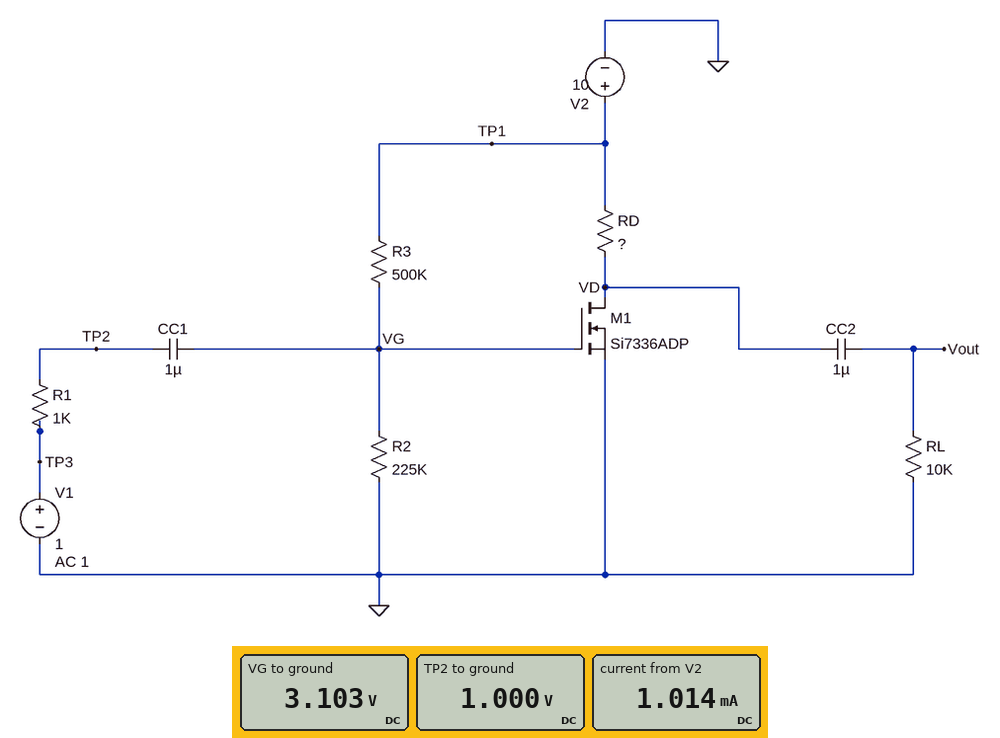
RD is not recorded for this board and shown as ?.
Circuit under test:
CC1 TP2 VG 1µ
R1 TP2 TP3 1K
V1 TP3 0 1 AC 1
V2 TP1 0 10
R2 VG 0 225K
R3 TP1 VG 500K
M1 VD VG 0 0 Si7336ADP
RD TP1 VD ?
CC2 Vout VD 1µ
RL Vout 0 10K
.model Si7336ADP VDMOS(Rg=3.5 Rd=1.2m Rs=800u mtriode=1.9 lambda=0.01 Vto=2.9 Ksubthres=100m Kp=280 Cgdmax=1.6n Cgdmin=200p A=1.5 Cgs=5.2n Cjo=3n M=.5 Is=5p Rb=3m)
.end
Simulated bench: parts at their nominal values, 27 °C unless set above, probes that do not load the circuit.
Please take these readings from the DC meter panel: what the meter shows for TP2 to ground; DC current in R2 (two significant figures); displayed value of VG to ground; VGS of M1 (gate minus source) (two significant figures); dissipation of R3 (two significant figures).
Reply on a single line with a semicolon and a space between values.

1.000 V; 14 µA; 3.103 V; 3.1 V; 95 µW
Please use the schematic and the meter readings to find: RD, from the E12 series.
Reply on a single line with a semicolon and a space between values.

10 kΩ
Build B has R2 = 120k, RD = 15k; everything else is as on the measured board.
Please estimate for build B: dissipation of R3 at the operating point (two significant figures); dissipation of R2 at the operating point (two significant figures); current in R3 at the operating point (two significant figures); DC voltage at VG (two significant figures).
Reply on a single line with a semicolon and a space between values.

130 µW; 31 µW; 16 µA; 1.9 V
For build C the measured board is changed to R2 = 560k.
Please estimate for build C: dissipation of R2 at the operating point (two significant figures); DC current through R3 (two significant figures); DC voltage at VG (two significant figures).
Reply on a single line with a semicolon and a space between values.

50 µW; 9.4 µA; 5.3 V
